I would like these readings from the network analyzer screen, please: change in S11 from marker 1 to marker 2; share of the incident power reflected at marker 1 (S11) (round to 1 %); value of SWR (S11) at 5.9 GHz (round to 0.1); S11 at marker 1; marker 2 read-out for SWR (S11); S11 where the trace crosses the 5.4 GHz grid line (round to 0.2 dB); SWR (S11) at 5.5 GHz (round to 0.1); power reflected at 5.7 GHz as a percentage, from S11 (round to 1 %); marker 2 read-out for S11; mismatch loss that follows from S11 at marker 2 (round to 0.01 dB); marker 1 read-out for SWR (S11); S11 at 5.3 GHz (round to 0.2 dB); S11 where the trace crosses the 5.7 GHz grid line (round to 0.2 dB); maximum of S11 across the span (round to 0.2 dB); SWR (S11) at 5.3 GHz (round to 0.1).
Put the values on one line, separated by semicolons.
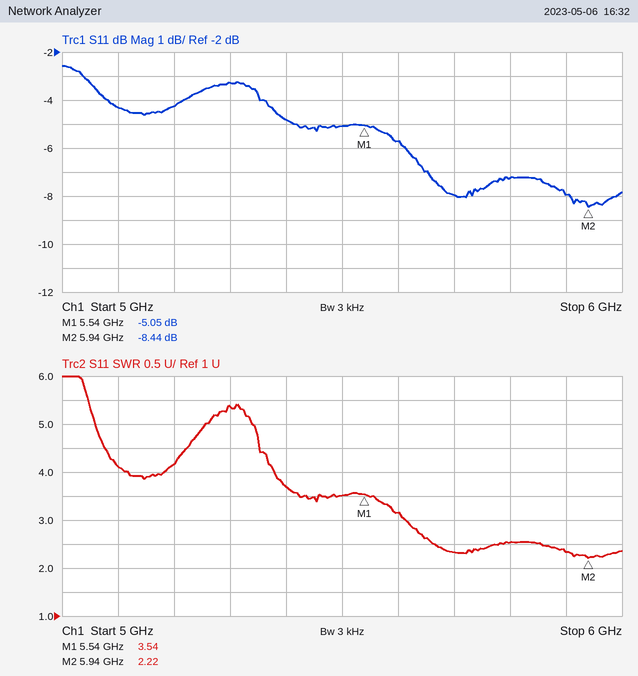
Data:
-3.39 dB; 31 %; 2.3; -5.05 dB; 2.22; -4.8 dB; 3.5; 16 %; -8.44 dB; 0.67 dB; 3.54; -3.2 dB; -8.0 dB; -2.6 dB; 5.4
